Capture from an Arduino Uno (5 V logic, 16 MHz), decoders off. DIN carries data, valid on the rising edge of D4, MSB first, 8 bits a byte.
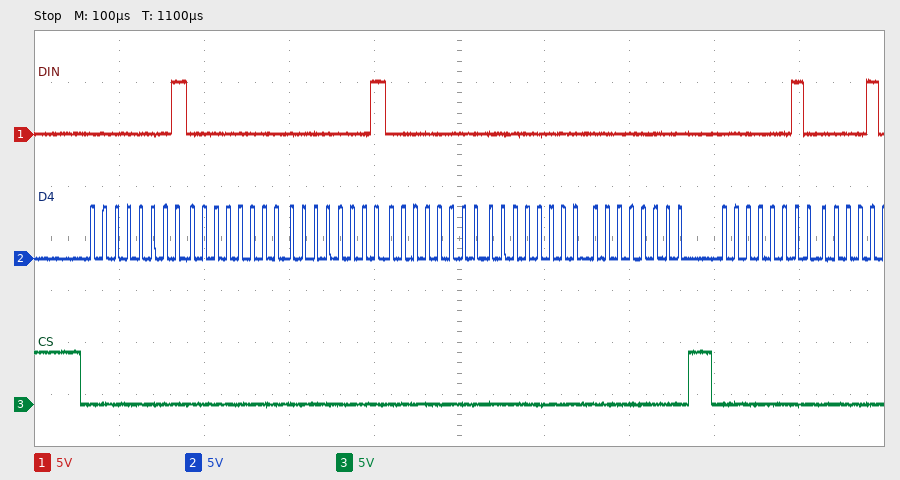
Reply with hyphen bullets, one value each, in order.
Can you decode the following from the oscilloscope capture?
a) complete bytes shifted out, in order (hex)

- 01 00 01 00 00 00 02
